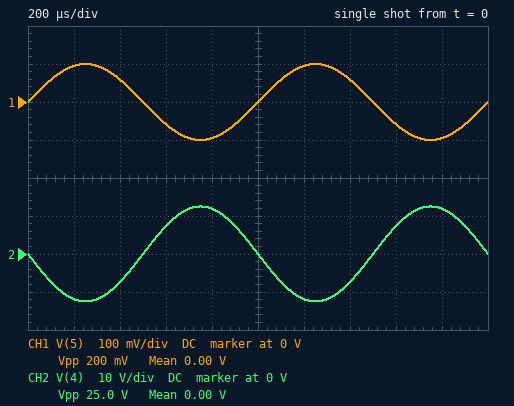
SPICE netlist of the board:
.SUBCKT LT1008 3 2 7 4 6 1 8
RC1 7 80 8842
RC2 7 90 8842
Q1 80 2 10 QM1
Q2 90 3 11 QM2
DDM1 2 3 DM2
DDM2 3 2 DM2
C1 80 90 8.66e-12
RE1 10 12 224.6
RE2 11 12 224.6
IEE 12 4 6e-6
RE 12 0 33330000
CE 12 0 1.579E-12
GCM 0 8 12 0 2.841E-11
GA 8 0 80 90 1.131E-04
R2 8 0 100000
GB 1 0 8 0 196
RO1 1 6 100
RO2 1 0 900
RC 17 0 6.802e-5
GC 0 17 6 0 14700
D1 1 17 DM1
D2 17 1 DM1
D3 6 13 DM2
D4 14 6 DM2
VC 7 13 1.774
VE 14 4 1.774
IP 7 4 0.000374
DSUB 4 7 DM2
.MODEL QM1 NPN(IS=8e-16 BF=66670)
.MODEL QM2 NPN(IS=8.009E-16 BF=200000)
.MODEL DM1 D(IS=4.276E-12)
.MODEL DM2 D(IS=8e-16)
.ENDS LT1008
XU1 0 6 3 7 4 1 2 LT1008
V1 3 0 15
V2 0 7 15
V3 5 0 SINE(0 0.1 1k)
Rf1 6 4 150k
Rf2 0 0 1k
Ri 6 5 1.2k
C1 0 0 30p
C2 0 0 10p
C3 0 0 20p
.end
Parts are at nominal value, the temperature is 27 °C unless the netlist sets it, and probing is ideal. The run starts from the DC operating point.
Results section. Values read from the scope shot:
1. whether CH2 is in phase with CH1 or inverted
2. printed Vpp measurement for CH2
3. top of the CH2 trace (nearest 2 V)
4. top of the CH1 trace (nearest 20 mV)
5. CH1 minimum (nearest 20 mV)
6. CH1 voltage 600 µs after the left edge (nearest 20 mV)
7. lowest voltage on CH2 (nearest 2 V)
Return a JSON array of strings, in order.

["inverted", "25.0 V", "12 V", "100 mV", "-100 mV", "-60 mV", "-12 V"]
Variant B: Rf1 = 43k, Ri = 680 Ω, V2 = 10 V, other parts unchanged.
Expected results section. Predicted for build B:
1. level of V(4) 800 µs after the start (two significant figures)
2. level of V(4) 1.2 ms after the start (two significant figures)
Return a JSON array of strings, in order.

["6.0 V", "-6.0 V"]
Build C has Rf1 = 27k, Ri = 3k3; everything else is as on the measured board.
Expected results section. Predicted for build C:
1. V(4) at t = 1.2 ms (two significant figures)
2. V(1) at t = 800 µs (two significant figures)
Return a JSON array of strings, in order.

["-780 mV", "780 mV"]
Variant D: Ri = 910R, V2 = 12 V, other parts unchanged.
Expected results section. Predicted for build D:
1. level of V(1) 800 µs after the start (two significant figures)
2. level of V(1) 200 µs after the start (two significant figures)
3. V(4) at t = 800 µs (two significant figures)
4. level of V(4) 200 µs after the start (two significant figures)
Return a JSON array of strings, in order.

["15 V", "-12 V", "14 V", "-11 V"]
